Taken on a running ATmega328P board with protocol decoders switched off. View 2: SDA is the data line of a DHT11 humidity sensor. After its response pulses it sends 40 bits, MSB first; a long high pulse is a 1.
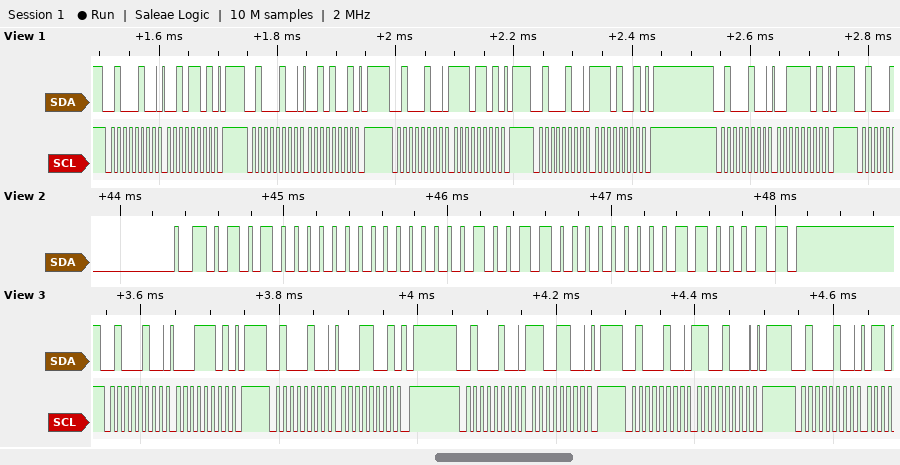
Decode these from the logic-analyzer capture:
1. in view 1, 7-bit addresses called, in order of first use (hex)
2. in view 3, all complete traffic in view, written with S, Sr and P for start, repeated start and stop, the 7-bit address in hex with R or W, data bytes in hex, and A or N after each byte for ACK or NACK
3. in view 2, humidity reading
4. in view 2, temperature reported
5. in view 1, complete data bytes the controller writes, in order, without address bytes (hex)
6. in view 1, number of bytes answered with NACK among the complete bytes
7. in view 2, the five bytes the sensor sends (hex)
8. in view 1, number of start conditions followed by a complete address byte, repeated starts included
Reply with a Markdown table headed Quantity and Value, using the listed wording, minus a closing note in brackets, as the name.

| Quantity | Value |
|---|---|
| in view 1, 7-bit addresses called, in order of first use | 0x22 |
| in view 3, all complete traffic in view, written with S, Sr and P for start, repeated start and stop, the 7-bit address in hex with R or W, data bytes in hex, and A or N after each byte for ACK or NACK | S 22W A 1D A P S 22W A 19 A P S 22W A CC A P S 22W A C8 A P S 22W A |
| in view 2, humidity reading | 80 % |
| in view 2, temperature reported | 19.0 °C |
| in view 1, complete data bytes the controller writes, in order, without address bytes | 2D 29 ED E9 3D |
| in view 1, number of bytes answered with NACK among the complete bytes | 0 |
| in view 2, the five bytes the sensor sends | 50 00 13 00 63 |
| in view 1, number of start conditions followed by a complete address byte, repeated starts included | 5 |
